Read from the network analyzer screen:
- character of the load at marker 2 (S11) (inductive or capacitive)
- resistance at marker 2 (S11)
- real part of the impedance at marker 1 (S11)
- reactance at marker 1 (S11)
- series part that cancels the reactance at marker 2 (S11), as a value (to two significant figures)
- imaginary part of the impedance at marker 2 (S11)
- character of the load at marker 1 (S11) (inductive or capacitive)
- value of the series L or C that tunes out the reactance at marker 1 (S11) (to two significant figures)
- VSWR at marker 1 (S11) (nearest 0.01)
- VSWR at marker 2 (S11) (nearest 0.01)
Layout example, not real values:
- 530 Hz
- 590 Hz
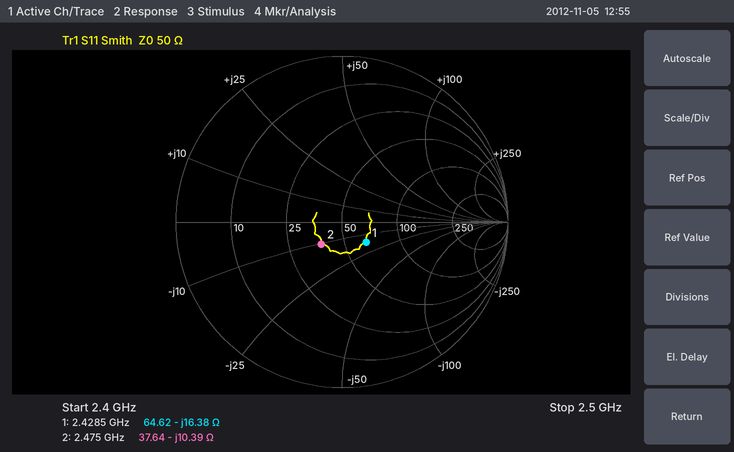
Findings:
- capacitive
- 37.64 Ω
- 64.62 Ω
- -16.38 Ω
- 670 pH
- -10.39 Ω
- capacitive
- 1.1 nH
- 1.47
- 1.45
